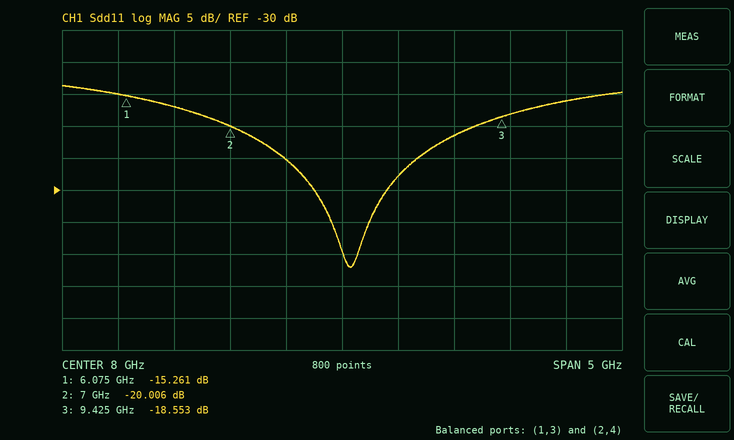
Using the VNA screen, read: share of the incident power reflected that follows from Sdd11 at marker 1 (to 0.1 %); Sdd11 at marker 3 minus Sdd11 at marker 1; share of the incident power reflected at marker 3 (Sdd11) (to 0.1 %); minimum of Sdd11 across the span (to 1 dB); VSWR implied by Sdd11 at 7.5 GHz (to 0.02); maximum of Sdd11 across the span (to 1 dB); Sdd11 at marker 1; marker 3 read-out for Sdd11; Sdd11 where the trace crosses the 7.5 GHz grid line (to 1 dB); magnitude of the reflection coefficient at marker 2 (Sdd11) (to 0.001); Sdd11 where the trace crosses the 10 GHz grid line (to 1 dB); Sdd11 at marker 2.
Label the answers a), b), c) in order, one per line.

a) 3.0 %
b) -3.292 dB
c) 1.4 %
d) -42 dB
e) 1.12
f) -14 dB
g) -15.261 dB
h) -18.553 dB
i) -25 dB
j) 0.100
k) -16 dB
l) -20.006 dB
